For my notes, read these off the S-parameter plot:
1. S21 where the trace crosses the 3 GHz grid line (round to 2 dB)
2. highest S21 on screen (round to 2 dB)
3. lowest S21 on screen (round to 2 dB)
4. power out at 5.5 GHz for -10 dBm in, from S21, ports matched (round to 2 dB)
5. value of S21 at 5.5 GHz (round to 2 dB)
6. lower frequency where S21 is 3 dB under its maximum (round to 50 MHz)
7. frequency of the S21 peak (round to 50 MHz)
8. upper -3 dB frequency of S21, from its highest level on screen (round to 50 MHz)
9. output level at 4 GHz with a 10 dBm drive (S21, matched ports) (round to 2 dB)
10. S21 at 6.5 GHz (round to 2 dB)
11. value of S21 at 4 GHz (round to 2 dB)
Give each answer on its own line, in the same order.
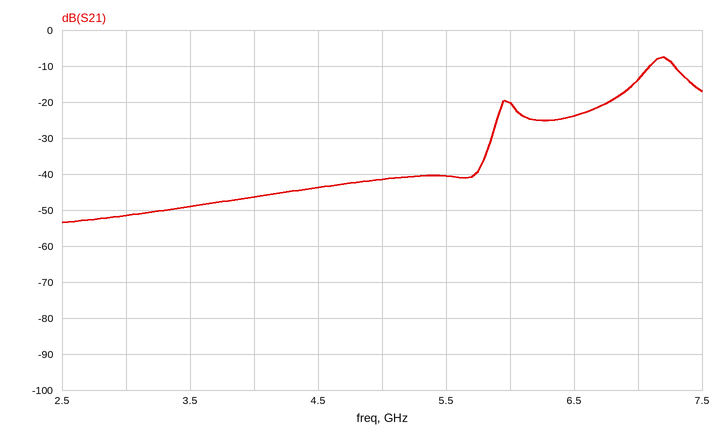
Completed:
-52 dB
-8 dB
-54 dB
-50 dBm
-40 dB
7.10 GHz
7.20 GHz
7.30 GHz
-36 dBm
-24 dB
-46 dB
